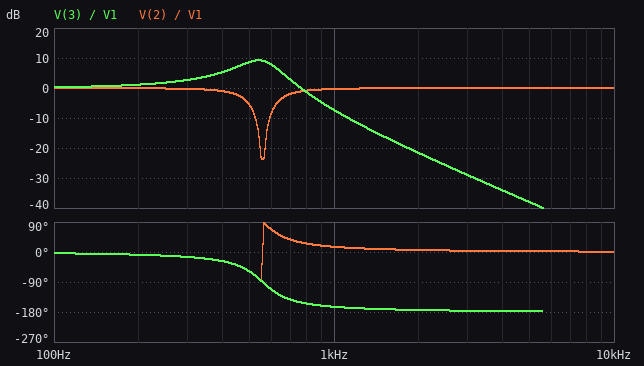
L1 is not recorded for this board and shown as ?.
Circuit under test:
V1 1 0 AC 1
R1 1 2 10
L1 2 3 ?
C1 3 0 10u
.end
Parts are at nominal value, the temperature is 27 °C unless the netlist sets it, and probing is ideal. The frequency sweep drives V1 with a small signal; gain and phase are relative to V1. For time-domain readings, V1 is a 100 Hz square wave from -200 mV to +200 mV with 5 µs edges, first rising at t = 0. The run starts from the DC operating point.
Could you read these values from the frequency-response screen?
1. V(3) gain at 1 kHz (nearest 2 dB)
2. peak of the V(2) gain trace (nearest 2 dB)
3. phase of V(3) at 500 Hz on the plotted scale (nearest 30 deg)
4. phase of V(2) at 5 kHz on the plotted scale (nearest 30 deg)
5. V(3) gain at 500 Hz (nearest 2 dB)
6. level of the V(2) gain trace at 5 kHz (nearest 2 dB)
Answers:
-8 dB
0 dB
-60 deg
0 deg
8 dB
0 dB
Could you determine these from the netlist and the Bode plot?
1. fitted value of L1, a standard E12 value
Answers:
8.2 mH
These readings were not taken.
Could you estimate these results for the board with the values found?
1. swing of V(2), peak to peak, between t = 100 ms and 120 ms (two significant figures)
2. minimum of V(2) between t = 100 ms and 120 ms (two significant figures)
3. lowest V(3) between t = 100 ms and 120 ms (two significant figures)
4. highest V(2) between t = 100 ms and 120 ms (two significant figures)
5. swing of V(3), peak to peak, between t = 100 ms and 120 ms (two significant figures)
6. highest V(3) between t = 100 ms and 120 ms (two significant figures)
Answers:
530 mV
-260 mV
-430 mV
260 mV
860 mV
430 mV
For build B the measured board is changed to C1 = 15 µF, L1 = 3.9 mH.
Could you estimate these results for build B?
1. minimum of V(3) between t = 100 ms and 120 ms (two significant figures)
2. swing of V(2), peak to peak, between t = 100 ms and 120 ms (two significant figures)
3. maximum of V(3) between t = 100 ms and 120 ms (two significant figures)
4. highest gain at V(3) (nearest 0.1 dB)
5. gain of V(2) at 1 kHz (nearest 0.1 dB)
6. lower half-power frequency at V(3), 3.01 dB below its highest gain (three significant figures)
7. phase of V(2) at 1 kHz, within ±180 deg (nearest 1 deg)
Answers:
-340 mV
520 mV
340 mV
4.6 dB
-1.8 dB
307 Hz
36 deg
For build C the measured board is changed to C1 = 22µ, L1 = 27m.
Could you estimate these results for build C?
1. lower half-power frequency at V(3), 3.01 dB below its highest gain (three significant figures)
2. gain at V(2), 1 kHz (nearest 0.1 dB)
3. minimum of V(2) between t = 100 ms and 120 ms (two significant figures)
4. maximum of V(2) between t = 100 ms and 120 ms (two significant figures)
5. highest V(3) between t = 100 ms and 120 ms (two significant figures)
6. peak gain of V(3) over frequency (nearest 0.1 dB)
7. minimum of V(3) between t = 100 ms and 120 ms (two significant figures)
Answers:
170 Hz
0 dB
-240 mV
240 mV
380 mV
11.0 dB
-380 mV
